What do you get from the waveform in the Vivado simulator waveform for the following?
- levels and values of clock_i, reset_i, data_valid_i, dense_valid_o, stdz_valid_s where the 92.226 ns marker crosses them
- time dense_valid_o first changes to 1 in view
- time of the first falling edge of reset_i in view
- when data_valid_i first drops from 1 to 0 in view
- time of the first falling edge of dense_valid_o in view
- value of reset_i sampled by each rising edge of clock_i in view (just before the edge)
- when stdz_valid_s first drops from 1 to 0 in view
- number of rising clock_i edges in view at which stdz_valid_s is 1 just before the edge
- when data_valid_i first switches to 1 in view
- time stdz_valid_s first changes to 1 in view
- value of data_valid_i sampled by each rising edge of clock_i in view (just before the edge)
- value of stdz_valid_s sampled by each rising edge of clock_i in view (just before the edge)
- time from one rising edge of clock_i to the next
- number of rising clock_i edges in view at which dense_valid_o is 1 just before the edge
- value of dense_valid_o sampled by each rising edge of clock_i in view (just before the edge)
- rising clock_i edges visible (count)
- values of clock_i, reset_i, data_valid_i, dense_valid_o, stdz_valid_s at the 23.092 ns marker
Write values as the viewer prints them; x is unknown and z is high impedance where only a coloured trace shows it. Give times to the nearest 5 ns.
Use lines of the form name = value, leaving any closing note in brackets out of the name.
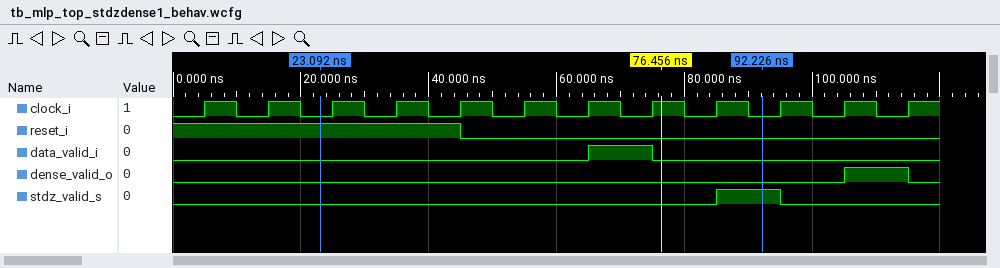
levels and values of clock_i, reset_i, data_valid_i, dense_valid_o, stdz_valid_s where the 92.226 ns marker crosses them = clock_i=0, reset_i=0, data_valid_i=0, dense_valid_o=0, stdz_valid_s=1
time dense_valid_o first changes to 1 in view = 105 ns
time of the first falling edge of reset_i in view = 45 ns
when data_valid_i first drops from 1 to 0 in view = 75 ns
time of the first falling edge of dense_valid_o in view = 115 ns
value of reset_i sampled by each rising edge of clock_i in view = 1 1 1 1 1 0 0 0 0 0 0 0
when stdz_valid_s first drops from 1 to 0 in view = 95 ns
number of rising clock_i edges in view at which stdz_valid_s is 1 just before the edge = 1
when data_valid_i first switches to 1 in view = 65 ns
time stdz_valid_s first changes to 1 in view = 85 ns
value of data_valid_i sampled by each rising edge of clock_i in view = 0 0 0 0 0 0 0 1 0 0 0 0
value of stdz_valid_s sampled by each rising edge of clock_i in view = 0 0 0 0 0 0 0 0 0 1 0 0
time from one rising edge of clock_i to the next = 10 ns
number of rising clock_i edges in view at which dense_valid_o is 1 just before the edge = 1
value of dense_valid_o sampled by each rising edge of clock_i in view = 0 0 0 0 0 0 0 0 0 0 0 1
rising clock_i edges visible = 12
values of clock_i, reset_i, data_valid_i, dense_valid_o, stdz_valid_s at the 23.092 ns marker = clock_i=0, reset_i=1, data_valid_i=0, dense_valid_o=0, stdz_valid_s=0
